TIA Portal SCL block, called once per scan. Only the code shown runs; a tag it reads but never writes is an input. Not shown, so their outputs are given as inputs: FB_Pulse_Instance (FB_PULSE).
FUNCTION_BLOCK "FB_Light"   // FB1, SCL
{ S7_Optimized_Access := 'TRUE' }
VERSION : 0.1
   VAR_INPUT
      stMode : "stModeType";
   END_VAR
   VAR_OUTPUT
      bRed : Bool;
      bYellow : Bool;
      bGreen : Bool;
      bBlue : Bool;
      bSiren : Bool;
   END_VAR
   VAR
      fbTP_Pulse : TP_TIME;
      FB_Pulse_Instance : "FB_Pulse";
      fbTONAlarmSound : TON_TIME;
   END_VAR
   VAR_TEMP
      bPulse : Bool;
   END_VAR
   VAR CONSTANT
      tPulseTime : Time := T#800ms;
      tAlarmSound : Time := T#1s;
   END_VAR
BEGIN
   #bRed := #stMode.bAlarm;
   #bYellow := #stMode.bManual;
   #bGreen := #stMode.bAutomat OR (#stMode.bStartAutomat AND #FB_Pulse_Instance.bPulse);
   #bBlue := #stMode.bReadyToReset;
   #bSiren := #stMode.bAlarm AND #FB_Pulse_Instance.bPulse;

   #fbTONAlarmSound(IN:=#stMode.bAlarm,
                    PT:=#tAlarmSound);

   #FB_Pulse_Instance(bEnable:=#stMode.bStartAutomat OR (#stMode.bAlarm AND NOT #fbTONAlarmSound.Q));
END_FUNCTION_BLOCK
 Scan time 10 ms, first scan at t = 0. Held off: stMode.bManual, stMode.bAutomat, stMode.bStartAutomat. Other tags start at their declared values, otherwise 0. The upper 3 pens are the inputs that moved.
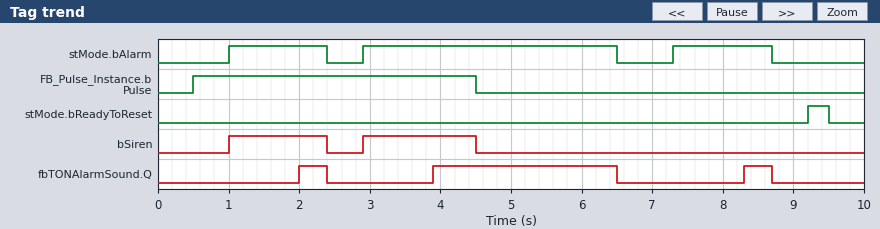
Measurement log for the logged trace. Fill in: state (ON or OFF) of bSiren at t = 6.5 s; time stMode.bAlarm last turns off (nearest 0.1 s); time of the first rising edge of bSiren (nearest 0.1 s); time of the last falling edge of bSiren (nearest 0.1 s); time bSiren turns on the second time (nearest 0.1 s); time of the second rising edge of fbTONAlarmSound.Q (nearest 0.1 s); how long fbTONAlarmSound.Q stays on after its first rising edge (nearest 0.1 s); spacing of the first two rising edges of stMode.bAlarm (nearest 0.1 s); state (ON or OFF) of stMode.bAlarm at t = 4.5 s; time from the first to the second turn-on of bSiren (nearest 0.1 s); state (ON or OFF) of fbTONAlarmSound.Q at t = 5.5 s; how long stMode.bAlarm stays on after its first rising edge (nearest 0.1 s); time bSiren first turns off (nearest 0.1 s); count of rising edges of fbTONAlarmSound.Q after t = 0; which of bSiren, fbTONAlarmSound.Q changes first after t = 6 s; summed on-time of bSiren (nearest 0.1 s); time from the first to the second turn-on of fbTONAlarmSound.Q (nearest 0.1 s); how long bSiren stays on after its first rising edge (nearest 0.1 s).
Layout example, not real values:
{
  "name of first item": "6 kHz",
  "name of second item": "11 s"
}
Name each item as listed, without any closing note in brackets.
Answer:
{
  "state (ON or OFF) of bSiren at t = 6.5 s": "OFF",
  "time stMode.bAlarm last turns off": "8.7 s",
  "time of the first rising edge of bSiren": "1.0 s",
  "time of the last falling edge of bSiren": "4.5 s",
  "time bSiren turns on the second time": "2.9 s",
  "time of the second rising edge of fbTONAlarmSound.Q": "3.9 s",
  "how long fbTONAlarmSound.Q stays on after its first rising edge": "0.4 s",
  "spacing of the first two rising edges of stMode.bAlarm": "1.9 s",
  "state (ON or OFF) of stMode.bAlarm at t = 4.5 s": "ON",
  "time from the first to the second turn-on of bSiren": "1.9 s",
  "state (ON or OFF) of fbTONAlarmSound.Q at t = 5.5 s": "ON",
  "how long stMode.bAlarm stays on after its first rising edge": "1.4 s",
  "time bSiren first turns off": "2.4 s",
  "count of rising edges of fbTONAlarmSound.Q after t = 0": "3",
  "which of bSiren, fbTONAlarmSound.Q changes first after t = 6 s": "fbTONAlarmSound.Q",
  "summed on-time of bSiren": "3.0 s",
  "time from the first to the second turn-on of fbTONAlarmSound.Q": "1.9 s",
  "how long bSiren stays on after its first rising edge": "1.4 s"
}
